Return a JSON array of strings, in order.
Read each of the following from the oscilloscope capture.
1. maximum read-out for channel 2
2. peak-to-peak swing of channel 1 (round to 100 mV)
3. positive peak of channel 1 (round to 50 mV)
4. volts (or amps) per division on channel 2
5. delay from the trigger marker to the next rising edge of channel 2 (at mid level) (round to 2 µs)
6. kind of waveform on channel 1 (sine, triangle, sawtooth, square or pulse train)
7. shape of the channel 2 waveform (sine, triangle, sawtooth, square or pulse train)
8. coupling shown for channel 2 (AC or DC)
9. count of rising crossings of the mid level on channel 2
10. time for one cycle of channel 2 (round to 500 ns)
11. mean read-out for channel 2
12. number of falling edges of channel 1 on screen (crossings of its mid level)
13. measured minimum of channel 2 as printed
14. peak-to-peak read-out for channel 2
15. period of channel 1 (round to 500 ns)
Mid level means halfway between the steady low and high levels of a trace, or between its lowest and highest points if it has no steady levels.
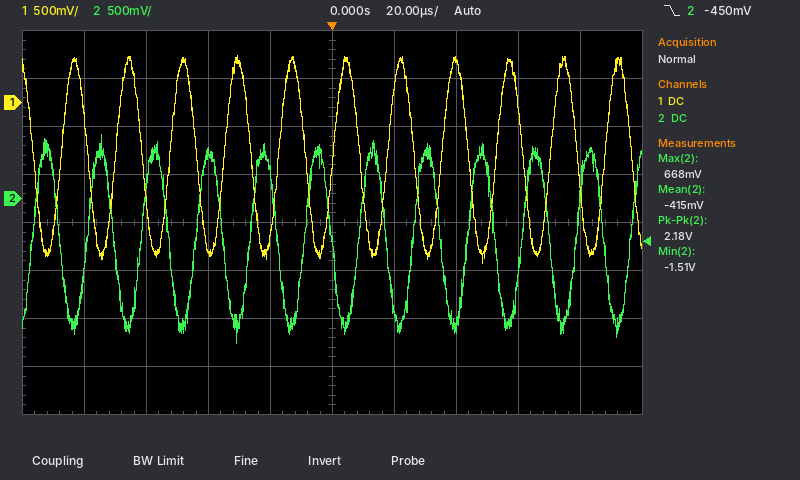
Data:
["668 mV", "2.20 V", "500 mV", "500 mV", "8 µs", "sine", "sine", "DC", "12", "17.5 µs", "-415 mV", "12", "-1.51 V", "2.18 V", "17.5 µs"]
